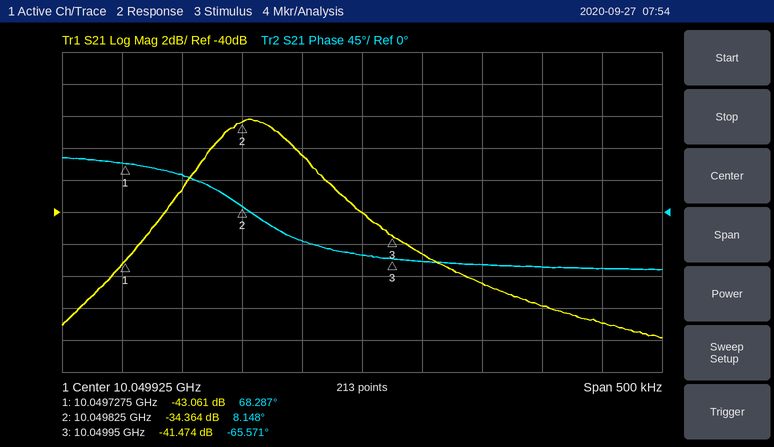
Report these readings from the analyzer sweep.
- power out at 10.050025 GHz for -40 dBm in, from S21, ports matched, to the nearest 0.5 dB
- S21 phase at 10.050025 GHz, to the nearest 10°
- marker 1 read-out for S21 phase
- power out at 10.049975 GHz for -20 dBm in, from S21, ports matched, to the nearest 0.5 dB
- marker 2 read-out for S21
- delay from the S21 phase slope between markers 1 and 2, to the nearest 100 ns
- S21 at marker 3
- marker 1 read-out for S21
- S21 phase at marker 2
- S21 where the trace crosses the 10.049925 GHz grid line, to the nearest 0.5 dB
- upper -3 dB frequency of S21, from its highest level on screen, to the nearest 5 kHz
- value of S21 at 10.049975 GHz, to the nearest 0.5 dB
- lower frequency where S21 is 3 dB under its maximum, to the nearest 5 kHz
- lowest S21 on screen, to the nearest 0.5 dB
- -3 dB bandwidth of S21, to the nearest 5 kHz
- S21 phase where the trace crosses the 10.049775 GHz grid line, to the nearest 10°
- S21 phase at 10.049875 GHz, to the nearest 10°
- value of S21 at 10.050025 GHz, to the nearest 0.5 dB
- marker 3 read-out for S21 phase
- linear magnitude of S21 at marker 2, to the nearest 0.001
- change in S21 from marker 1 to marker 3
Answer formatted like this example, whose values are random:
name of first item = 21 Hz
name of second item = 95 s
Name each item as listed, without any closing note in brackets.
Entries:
power out at 10.050025 GHz for -40 dBm in, from S21, ports matched, to the nearest 0.5 dB = -84.5 dBm
S21 phase at 10.050025 GHz, to the nearest 10° = -70°
marker 1 read-out for S21 phase = 68.287°
power out at 10.049975 GHz for -20 dBm in, from S21, ports matched, to the nearest 0.5 dB = -62.5 dBm
marker 2 read-out for S21 = -34.364 dB
delay from the S21 phase slope between markers 1 and 2, to the nearest 100 ns = 1.7 µs
S21 at marker 3 = -41.474 dB
marker 1 read-out for S21 = -43.061 dB
S21 phase at marker 2 = 8.148°
S21 where the trace crosses the 10.049925 GHz grid line, to the nearest 0.5 dB = -40.0 dB
upper -3 dB frequency of S21, from its highest level on screen, to the nearest 5 kHz = 10.049885 GHz
value of S21 at 10.049975 GHz, to the nearest 0.5 dB = -42.5 dB
lower frequency where S21 is 3 dB under its maximum, to the nearest 5 kHz = 10.049790 GHz
lowest S21 on screen, to the nearest 0.5 dB = -48.0 dB
-3 dB bandwidth of S21, to the nearest 5 kHz = 95 kHz
S21 phase where the trace crosses the 10.049775 GHz grid line, to the nearest 10° = 50°
S21 phase at 10.049875 GHz, to the nearest 10° = -40°
value of S21 at 10.050025 GHz, to the nearest 0.5 dB = -44.5 dB
marker 3 read-out for S21 phase = -65.571°
linear magnitude of S21 at marker 2, to the nearest 0.001 = 0.019
change in S21 from marker 1 to marker 3 = 1.587 dB
